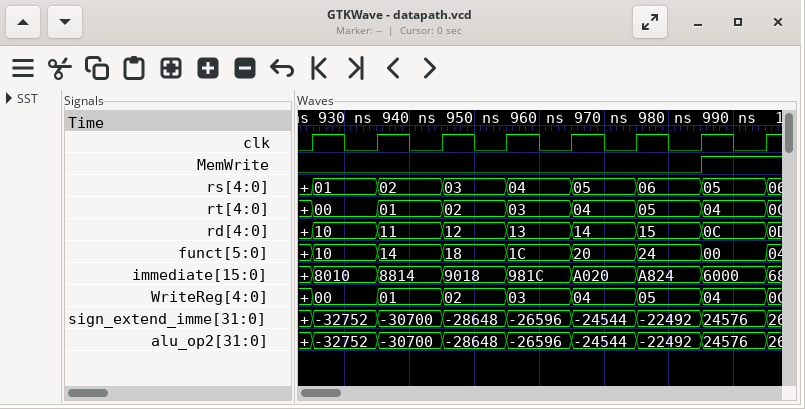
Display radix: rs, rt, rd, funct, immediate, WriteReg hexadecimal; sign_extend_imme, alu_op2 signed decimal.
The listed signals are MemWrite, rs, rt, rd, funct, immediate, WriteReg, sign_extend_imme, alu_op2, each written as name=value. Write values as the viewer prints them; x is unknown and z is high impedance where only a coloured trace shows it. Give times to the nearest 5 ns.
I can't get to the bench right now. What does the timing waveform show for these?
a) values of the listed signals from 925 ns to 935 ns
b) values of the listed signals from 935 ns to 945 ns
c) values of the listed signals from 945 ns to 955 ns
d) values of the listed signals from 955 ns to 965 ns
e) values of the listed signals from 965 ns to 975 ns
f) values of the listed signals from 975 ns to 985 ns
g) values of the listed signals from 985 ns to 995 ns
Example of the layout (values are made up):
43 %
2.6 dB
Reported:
MemWrite=0, rs=01, rt=00, rd=10, funct=10, immediate=8010, WriteReg=00, sign_extend_imme=-32752, alu_op2=-32752
MemWrite=0, rs=02, rt=01, rd=11, funct=14, immediate=8814, WriteReg=01, sign_extend_imme=-30700, alu_op2=-30700
MemWrite=0, rs=03, rt=02, rd=12, funct=18, immediate=9018, WriteReg=02, sign_extend_imme=-28648, alu_op2=-28648
MemWrite=0, rs=04, rt=03, rd=13, funct=1C, immediate=981C, WriteReg=03, sign_extend_imme=-26596, alu_op2=-26596
MemWrite=0, rs=05, rt=04, rd=14, funct=20, immediate=A020, WriteReg=04, sign_extend_imme=-24544, alu_op2=-24544
MemWrite=0, rs=06, rt=05, rd=15, funct=24, immediate=A824, WriteReg=05, sign_extend_imme=-22492, alu_op2=-22492
MemWrite=1, rs=05, rt=04, rd=0C, funct=00, immediate=6000, WriteReg=04, sign_extend_imme=24576, alu_op2=24576
